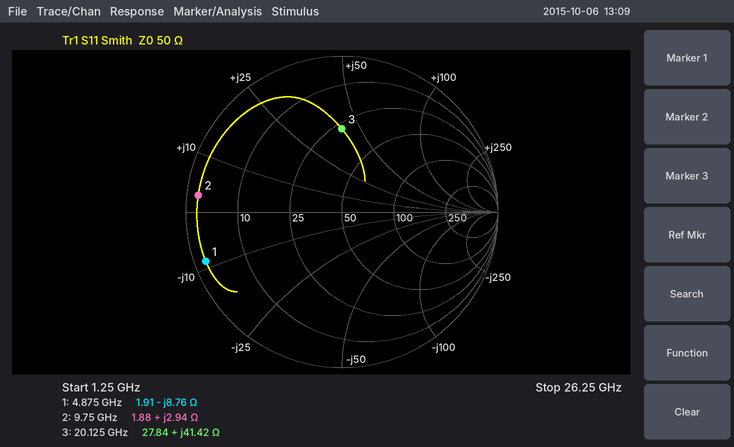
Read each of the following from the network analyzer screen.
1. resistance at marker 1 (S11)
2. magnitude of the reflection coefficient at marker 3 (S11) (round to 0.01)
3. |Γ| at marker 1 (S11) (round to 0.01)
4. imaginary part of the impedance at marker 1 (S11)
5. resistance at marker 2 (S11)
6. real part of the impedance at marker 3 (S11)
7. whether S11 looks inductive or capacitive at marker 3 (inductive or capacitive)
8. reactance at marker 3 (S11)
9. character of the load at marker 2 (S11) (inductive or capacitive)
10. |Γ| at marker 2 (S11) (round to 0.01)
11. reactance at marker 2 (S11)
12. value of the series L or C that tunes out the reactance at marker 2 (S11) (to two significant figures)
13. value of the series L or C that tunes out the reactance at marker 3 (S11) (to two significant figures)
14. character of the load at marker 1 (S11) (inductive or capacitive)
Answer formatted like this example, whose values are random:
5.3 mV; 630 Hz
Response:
1.91 Ω; 0.53; 0.93; -8.76 Ω; 1.88 Ω; 27.84 Ω; inductive; +41.42 Ω; inductive; 0.93; +2.94 Ω; 5.6 pF; 190 fF; capacitive
